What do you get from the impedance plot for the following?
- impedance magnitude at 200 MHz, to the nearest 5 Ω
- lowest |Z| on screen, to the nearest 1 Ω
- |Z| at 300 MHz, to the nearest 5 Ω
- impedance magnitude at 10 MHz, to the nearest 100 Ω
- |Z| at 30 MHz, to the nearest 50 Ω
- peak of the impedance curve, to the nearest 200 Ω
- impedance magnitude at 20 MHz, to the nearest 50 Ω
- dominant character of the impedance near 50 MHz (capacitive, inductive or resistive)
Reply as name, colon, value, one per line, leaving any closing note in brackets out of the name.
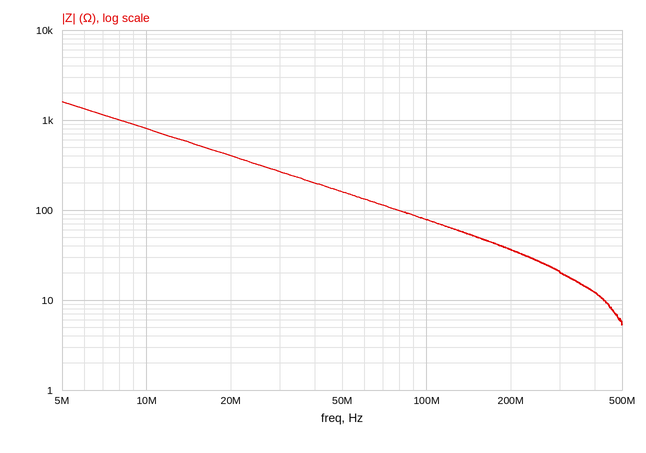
impedance magnitude at 200 MHz, to the nearest 5 Ω: 35 Ω
lowest |Z| on screen, to the nearest 1 Ω: 5 Ω
|Z| at 300 MHz, to the nearest 5 Ω: 20 Ω
impedance magnitude at 10 MHz, to the nearest 100 Ω: 800 Ω
|Z| at 30 MHz, to the nearest 50 Ω: 250 Ω
peak of the impedance curve, to the nearest 200 Ω: 1.6 kΩ
impedance magnitude at 20 MHz, to the nearest 50 Ω: 400 Ω
dominant character of the impedance near 50 MHz: capacitive
